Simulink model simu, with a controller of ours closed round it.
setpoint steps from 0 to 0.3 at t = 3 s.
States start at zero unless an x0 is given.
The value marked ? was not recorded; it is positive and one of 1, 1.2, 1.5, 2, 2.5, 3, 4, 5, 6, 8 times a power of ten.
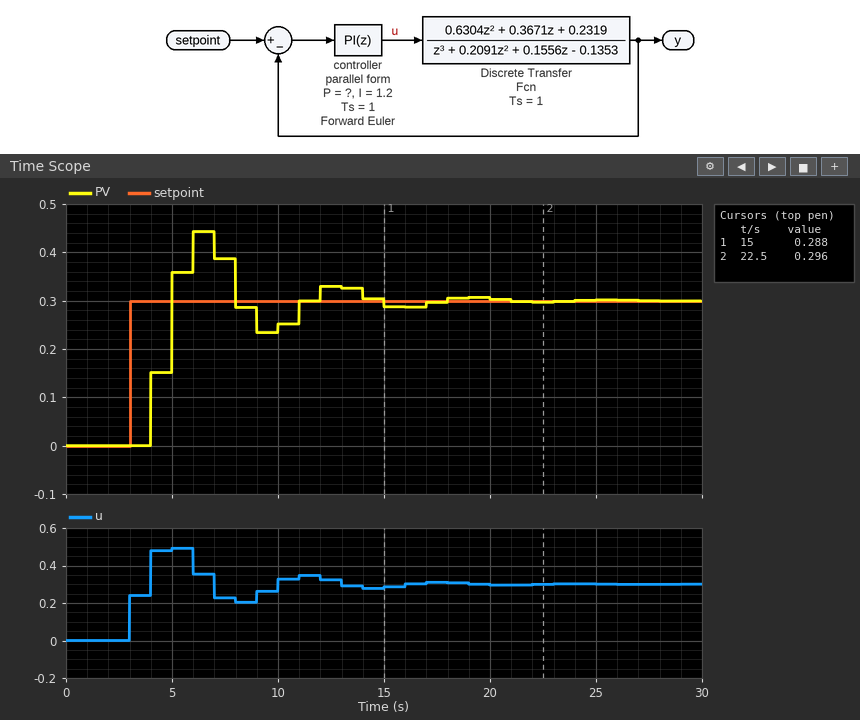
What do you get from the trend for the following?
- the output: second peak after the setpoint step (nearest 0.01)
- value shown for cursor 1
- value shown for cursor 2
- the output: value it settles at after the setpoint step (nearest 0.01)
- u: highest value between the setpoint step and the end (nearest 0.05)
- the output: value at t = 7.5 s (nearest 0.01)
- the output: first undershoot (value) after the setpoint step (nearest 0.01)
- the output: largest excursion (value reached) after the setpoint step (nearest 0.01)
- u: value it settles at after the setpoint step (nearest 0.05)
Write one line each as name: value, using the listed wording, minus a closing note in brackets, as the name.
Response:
the output: second peak after the setpoint step: 0.33
value shown for cursor 1: 0.288
value shown for cursor 2: 0.296
the output: value it settles at after the setpoint step: 0.30
u: highest value between the setpoint step and the end: 0.50
the output: value at t = 7.5 s: 0.39
the output: first undershoot (value) after the setpoint step: 0.23
the output: largest excursion (value reached) after the setpoint step: 0.44
u: value it settles at after the setpoint step: 0.30
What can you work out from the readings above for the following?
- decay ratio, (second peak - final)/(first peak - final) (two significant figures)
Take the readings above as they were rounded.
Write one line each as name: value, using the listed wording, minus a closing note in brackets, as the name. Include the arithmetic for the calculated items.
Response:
decay ratio, (second peak - final)/(first peak - final): (0.33 - 0.3) / (0.44 - 0.3) = 0.21
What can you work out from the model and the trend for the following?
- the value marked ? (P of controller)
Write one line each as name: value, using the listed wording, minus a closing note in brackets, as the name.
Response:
the value marked ?: 0.8
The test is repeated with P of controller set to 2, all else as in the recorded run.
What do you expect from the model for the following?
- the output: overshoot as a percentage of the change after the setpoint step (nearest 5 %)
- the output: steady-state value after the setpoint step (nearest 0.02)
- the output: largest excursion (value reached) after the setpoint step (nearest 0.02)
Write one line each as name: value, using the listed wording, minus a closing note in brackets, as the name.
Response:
the output: overshoot as a percentage of the change after the setpoint step: 25 %
the output: steady-state value after the setpoint step: 0.30
the output: largest excursion (value reached) after the setpoint step: 0.38
